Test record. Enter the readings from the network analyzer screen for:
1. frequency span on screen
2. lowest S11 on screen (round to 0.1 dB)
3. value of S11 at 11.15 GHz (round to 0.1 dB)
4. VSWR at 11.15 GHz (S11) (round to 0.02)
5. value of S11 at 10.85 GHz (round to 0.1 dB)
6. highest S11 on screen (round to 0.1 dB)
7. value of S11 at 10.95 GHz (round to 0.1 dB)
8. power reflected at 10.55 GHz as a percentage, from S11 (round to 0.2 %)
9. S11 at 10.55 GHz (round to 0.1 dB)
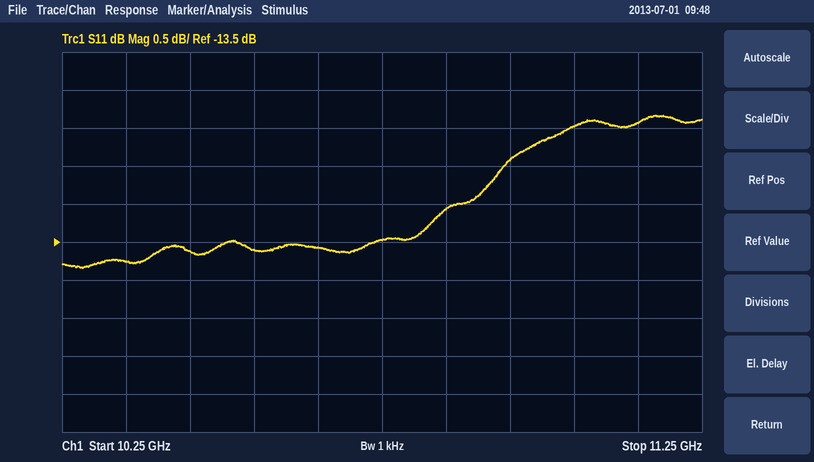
1 GHz
-13.8 dB
-11.9 dB
1.68
-13.1 dB
-11.8 dB
-12.4 dB
4.4 %
-13.6 dB
